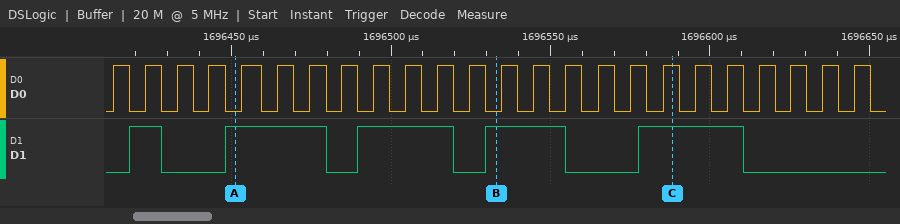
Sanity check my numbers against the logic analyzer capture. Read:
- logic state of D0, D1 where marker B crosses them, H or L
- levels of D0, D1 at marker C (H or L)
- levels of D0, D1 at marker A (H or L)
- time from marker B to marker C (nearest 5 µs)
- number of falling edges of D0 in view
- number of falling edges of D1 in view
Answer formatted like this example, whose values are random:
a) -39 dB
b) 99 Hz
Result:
a) D0=L, D1=H
b) D0=H, D1=H
c) D0=L, D1=H
d) 55 µs
e) 24
f) 5
